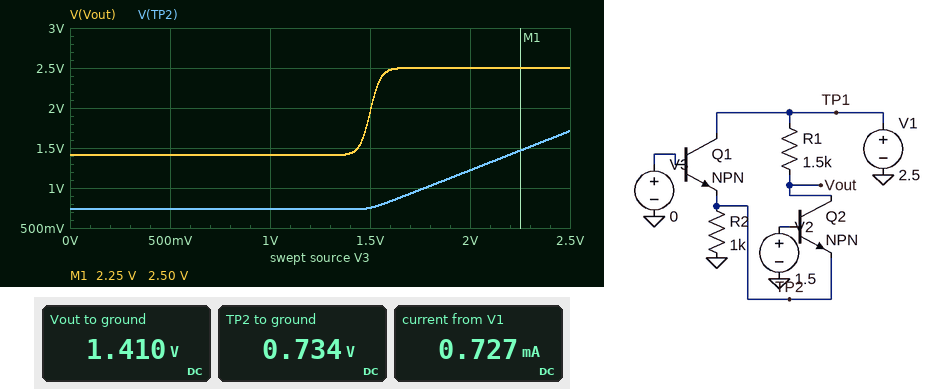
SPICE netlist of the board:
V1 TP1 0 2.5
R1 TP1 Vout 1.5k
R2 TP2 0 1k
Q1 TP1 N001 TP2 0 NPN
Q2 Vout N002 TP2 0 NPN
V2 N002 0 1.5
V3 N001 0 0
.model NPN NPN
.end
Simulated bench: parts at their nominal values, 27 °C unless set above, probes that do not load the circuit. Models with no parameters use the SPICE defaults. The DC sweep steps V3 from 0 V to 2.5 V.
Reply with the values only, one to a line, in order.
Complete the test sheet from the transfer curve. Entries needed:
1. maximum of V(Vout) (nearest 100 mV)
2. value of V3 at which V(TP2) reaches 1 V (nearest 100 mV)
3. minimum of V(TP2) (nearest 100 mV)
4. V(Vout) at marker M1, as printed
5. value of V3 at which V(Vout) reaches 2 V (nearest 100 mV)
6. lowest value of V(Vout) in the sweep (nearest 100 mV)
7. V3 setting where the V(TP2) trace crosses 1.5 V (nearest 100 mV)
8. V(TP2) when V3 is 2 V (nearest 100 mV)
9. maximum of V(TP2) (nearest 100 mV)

2.5 V
1.8 V
700 mV
2.50 V
1.5 V
1.4 V
2.3 V
1.2 V
1.7 V
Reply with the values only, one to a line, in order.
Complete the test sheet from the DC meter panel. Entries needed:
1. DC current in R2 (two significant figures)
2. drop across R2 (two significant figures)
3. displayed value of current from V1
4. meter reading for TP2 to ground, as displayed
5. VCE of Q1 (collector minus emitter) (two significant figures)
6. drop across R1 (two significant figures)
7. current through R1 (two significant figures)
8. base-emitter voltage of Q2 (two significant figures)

730 µA
730 mV
0.727 mA
0.734 V
1.8 V
1.1 V
730 µA
770 mV
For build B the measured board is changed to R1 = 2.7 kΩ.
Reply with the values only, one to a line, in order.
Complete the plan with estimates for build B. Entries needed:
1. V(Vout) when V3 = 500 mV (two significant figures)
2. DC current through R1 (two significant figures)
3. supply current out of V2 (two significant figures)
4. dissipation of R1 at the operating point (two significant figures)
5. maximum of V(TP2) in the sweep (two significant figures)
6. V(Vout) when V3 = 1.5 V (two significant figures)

790 mV
630 µA
97 µA
1.1 mW
1.7 V
1.5 V
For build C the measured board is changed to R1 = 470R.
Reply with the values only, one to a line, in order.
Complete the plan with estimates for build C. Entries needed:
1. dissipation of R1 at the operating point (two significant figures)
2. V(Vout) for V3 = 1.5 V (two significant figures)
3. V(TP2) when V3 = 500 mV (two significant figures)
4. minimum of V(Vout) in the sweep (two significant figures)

250 µW
2.3 V
730 mV
2.2 V
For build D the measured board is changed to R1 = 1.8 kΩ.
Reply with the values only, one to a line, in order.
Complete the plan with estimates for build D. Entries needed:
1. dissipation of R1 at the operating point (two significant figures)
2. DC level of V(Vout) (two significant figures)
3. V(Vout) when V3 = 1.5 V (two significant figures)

950 µW
1.2 V
1.8 V
